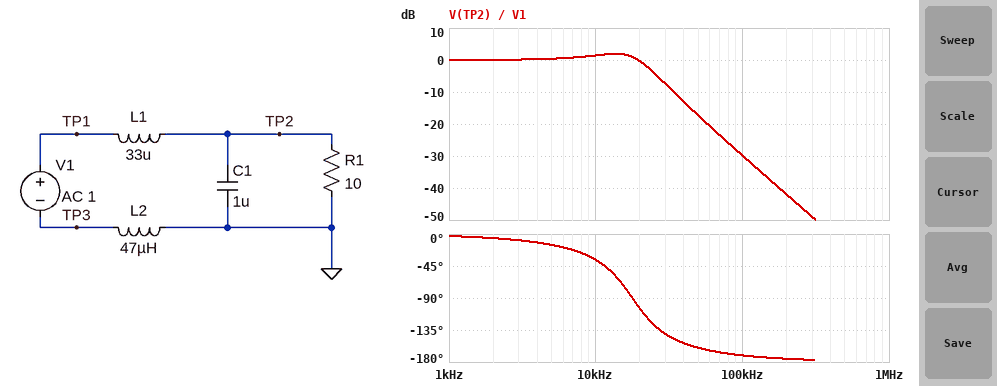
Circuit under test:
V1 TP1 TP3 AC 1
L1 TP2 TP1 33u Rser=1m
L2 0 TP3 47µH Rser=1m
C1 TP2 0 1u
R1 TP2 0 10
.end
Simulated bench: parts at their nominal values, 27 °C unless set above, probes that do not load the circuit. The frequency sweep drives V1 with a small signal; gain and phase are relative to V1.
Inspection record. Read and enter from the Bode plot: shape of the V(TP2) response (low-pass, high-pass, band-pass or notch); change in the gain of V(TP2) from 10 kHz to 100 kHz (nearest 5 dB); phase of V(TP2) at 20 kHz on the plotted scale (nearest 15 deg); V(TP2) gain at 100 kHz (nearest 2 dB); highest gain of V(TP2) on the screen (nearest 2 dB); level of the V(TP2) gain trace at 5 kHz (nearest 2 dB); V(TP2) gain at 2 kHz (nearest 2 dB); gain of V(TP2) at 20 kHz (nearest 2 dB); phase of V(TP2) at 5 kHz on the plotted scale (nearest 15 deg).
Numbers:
low-pass
-30 dB
-105 deg
-30 dB
2 dB
0 dB
0 dB
0 dB
-15 deg
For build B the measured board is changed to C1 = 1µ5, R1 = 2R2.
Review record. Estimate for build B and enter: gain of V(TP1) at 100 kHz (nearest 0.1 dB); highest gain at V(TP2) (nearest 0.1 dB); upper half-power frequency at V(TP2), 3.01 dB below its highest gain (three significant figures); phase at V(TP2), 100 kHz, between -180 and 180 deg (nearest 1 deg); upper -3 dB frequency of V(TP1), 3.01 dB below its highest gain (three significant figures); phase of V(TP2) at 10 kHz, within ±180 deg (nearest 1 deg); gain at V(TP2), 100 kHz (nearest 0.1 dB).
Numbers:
-7.9 dB
0 dB
4.81 kHz
-154 deg
5.49 kHz
-77 deg
-34.3 dB
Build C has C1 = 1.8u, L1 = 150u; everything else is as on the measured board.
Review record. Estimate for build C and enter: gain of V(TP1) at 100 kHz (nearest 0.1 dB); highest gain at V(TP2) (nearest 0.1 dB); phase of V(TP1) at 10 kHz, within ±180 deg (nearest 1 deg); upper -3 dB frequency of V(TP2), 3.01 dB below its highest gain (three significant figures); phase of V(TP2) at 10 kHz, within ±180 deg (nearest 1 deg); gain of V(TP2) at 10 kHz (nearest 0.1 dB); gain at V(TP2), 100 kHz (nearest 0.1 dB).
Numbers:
-2.4 dB
1.0 dB
-14 deg
9.80 kHz
-108 deg
-2.3 dB
-42.9 dB
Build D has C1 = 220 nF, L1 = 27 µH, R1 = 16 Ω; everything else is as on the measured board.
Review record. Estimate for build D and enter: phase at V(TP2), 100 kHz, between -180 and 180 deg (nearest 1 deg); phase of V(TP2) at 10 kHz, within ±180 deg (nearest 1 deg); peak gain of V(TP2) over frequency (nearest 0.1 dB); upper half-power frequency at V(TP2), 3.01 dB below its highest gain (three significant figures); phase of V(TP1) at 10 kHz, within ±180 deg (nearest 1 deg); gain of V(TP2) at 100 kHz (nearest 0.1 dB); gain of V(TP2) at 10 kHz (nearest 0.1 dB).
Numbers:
-152 deg
-17 deg
0.5 dB
44.7 kHz
-11 deg
-15.8 dB
0.2 dB
